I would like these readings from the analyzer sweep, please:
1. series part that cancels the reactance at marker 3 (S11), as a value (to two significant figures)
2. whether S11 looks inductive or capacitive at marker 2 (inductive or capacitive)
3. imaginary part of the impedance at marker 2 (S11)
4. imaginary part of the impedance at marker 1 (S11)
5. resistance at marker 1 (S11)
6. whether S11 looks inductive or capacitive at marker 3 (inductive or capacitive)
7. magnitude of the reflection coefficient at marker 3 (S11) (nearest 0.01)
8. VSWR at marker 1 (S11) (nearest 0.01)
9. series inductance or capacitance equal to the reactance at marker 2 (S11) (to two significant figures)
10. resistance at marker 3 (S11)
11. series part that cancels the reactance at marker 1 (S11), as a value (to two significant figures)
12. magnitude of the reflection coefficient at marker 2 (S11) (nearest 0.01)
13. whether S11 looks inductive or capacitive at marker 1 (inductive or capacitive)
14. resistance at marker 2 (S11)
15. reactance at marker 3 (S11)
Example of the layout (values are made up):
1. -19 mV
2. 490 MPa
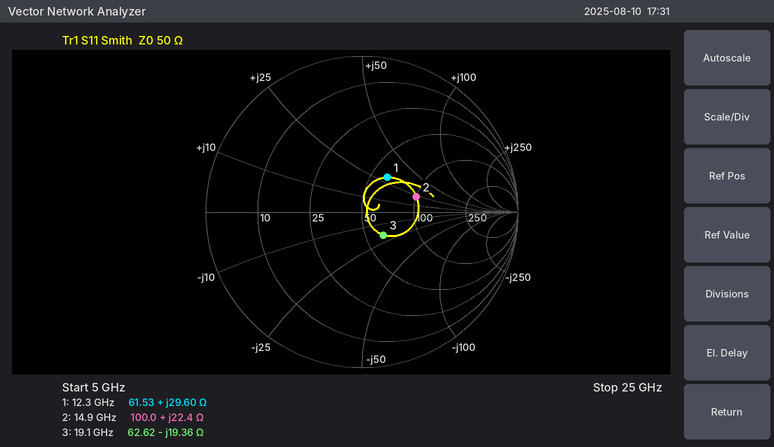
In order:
1. 160 pH
2. inductive
3. +22.4 Ω
4. +29.60 Ω
5. 61.53 Ω
6. capacitive
7. 0.20
8. 1.76
9. 240 pH
10. 62.62 Ω
11. 440 fF
12. 0.36
13. inductive
14. 100.0 Ω
15. -19.36 Ω
